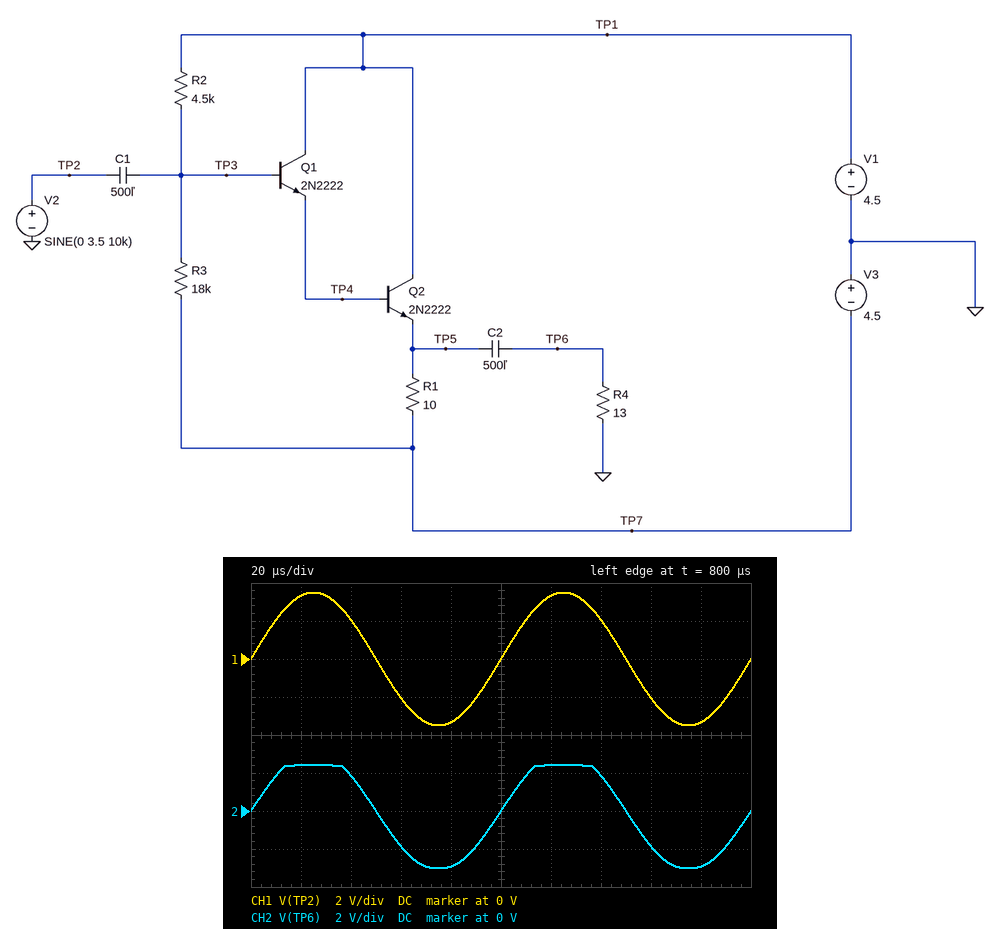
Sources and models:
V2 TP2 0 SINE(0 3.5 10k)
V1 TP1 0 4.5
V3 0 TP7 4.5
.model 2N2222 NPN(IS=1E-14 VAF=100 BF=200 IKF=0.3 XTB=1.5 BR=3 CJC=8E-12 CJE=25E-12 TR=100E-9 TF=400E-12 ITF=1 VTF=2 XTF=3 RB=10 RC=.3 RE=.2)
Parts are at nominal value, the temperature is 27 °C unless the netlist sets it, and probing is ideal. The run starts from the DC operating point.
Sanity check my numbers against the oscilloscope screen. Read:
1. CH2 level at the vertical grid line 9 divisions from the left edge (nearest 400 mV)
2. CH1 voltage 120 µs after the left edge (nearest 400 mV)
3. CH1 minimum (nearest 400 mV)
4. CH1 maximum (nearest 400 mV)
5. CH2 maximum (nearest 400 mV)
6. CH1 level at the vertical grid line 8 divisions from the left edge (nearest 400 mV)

-2.8 V
3.2 V
-3.6 V
3.6 V
2.4 V
-2.0 V
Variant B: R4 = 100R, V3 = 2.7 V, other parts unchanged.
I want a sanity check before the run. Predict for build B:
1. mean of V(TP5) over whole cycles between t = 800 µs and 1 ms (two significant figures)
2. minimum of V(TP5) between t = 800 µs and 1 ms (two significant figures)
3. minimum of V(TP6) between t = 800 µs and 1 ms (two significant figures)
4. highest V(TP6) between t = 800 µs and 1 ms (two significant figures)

1.1 V
-1.9 V
-3.2 V
2.1 V
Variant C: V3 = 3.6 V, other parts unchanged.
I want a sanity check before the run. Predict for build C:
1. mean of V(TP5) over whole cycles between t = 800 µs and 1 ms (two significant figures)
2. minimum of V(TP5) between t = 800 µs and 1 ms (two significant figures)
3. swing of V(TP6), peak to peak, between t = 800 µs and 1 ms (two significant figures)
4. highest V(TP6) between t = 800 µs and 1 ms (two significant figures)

1.0 V
-1.6 V
4.9 V
2.2 V
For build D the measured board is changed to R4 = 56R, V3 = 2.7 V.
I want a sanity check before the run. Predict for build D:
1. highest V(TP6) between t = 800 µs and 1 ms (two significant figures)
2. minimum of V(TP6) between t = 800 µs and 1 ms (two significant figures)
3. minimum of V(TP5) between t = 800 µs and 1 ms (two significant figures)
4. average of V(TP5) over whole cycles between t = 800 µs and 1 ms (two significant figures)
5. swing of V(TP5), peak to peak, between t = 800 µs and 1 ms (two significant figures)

2.1 V
-3.2 V
-1.9 V
1.1 V
5.3 V
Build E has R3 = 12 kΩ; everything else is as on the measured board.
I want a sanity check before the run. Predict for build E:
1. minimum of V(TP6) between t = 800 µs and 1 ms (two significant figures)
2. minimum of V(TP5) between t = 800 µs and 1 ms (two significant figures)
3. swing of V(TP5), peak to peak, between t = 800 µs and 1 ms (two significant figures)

-2.7 V
-2.4 V
5.6 V
